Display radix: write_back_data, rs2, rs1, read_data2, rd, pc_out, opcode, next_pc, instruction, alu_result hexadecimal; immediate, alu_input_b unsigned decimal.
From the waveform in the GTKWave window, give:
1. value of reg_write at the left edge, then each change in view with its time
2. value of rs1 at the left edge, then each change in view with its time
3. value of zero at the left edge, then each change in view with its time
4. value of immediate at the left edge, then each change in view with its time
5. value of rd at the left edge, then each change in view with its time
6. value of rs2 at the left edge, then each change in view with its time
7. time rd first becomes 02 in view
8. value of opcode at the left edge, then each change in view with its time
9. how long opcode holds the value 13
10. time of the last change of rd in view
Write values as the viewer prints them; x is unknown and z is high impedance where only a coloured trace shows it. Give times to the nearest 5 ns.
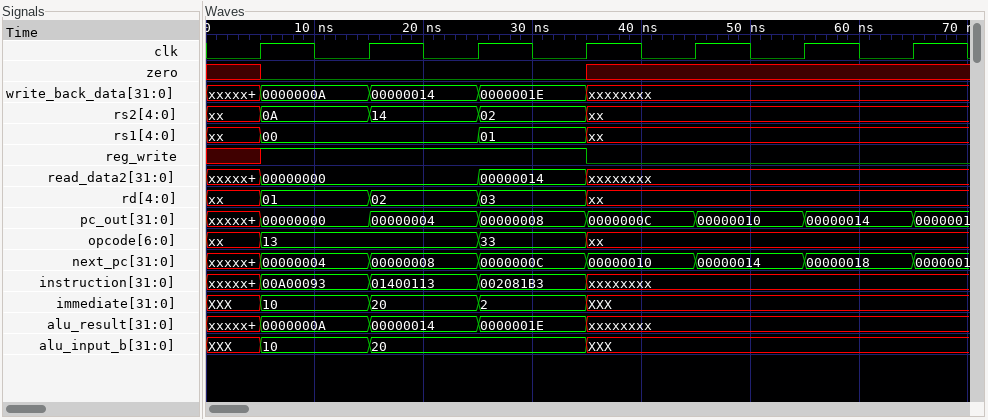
x, 1 at 5 ns, 0 at 35 ns
xx, 00 at 5 ns, 01 at 25 ns, xx at 35 ns
x, 0 at 5 ns, x at 35 ns
XXX, 10 at 5 ns, 20 at 15 ns, 2 at 25 ns, XXX at 35 ns
xx, 01 at 5 ns, 02 at 15 ns, 03 at 25 ns, xx at 35 ns
xx, 0A at 5 ns, 14 at 15 ns, 02 at 25 ns, xx at 35 ns
15 ns
xx, 13 at 5 ns, 33 at 25 ns, xx at 35 ns
20 ns
35 ns
